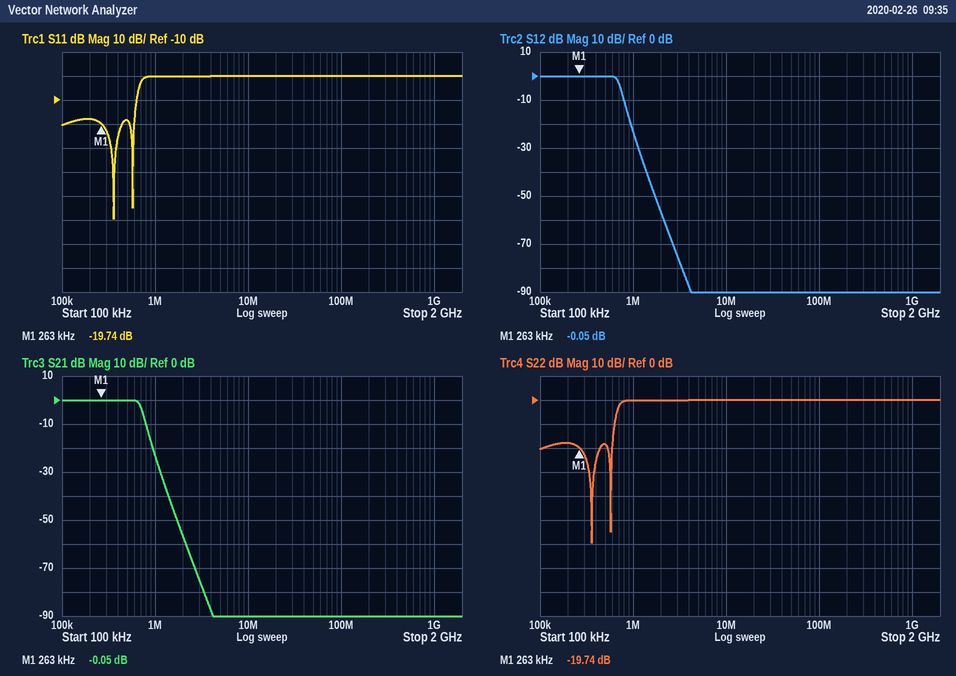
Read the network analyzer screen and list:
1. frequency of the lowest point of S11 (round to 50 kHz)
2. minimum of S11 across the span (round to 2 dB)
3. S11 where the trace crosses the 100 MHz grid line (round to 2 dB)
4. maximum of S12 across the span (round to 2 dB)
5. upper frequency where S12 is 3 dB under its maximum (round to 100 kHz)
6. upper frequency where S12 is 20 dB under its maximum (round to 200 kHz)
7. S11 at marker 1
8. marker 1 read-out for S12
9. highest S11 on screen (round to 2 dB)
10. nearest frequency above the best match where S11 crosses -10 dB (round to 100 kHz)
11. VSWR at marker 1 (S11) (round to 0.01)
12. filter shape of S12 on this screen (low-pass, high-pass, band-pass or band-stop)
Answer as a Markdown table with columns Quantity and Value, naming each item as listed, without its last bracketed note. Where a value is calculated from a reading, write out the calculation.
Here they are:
| Quantity | Value |
|---|---|
| frequency of the lowest point of S11 | 350 kHz |
| minimum of S11 across the span | -60 dB |
| S11 where the trace crosses the 100 MHz grid line | 0 dB |
| maximum of S12 across the span | 0 dB |
| upper frequency where S12 is 3 dB under its maximum | 700 kHz |
| upper frequency where S12 is 20 dB under its maximum | 1.0 MHz |
| S11 at marker 1 | -19.74 dB |
| marker 1 read-out for S12 | -0.05 dB |
| highest S11 on screen | 0 dB |
| nearest frequency above the best match where S11 crosses -10 dB | 600 kHz |
| VSWR at marker 1 (S11) | (1 + 0.1030)/(1 − 0.1030) ≈ 1.23 |
| filter shape of S12 on this screen | low-pass |
